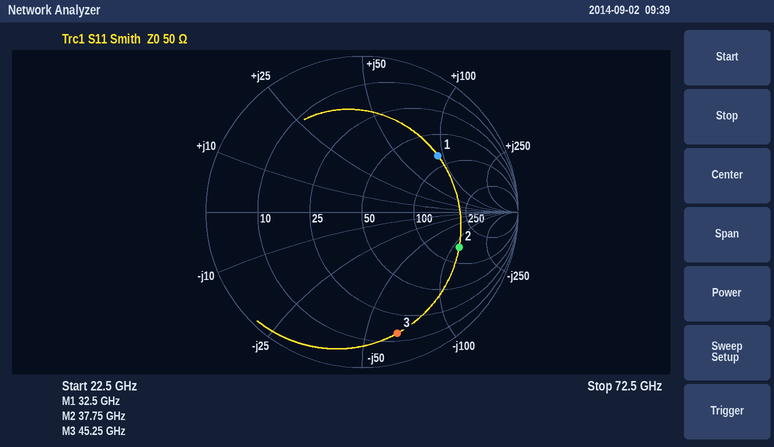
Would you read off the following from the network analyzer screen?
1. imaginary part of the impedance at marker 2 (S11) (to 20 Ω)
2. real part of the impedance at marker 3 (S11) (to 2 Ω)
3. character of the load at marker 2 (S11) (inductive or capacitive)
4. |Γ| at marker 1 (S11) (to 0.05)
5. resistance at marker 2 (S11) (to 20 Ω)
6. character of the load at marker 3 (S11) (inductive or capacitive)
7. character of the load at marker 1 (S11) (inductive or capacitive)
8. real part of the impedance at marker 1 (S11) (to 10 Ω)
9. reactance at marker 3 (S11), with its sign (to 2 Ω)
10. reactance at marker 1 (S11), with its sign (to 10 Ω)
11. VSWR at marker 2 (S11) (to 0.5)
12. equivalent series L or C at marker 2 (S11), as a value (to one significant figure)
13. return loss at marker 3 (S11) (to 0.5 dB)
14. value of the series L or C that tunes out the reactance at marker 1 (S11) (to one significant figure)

-120 Ω
14 Ω
capacitive
0.60
140 Ω
capacitive
inductive
80 Ω
-64 Ω
+90 Ω
5.0
40 fF
2.0 dB
50 fF
